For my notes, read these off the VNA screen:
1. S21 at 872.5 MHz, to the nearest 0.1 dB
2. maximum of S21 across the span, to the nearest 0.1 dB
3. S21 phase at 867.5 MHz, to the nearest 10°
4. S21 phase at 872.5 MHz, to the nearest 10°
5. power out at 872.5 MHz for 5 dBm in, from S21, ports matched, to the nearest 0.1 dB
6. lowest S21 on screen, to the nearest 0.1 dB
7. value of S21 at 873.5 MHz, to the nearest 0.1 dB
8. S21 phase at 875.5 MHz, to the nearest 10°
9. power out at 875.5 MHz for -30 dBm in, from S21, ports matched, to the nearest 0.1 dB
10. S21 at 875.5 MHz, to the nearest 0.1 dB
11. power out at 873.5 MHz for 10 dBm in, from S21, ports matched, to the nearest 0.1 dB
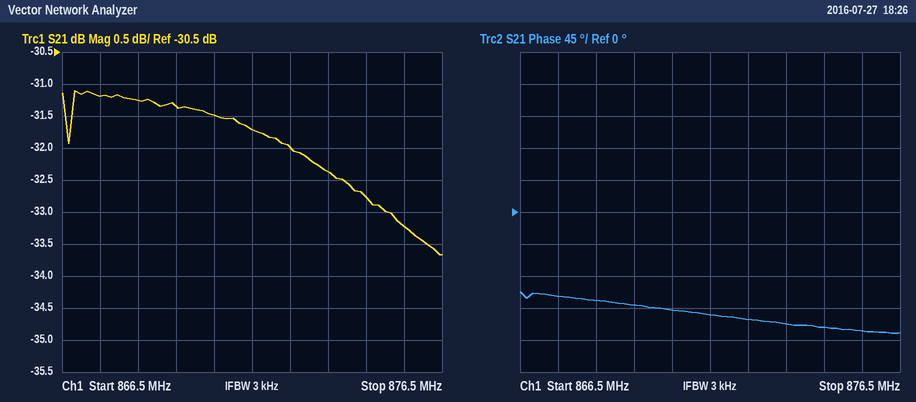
-32.0 dB
-31.1 dB
-120°
-150°
-27.0 dBm
-33.7 dB
-32.4 dB
-170°
-63.2 dBm
-33.2 dB
-22.4 dBm
